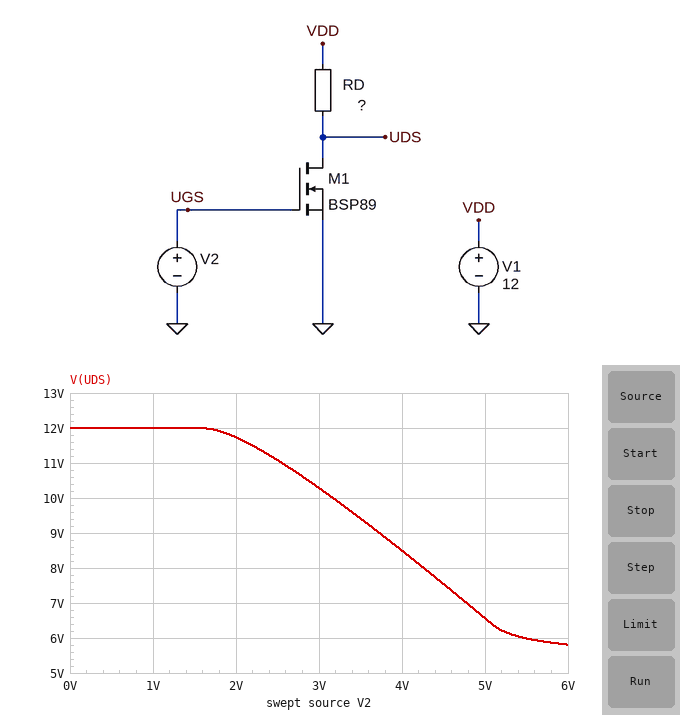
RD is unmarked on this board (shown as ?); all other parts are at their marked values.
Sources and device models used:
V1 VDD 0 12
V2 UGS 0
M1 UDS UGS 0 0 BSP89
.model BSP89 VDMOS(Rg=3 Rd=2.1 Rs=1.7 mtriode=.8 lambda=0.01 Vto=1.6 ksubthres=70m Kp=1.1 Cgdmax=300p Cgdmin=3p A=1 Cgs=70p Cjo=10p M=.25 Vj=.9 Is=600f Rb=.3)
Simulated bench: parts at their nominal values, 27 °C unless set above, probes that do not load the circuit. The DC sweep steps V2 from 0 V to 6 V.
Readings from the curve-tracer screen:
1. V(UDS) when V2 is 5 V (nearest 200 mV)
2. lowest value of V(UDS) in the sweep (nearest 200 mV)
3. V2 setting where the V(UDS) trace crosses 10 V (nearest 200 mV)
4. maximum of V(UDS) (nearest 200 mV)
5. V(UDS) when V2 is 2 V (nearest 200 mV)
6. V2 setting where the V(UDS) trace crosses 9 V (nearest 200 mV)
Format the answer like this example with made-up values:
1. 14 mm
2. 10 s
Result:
1. 6.6 V
2. 5.8 V
3. 3.2 V
4. 12.0 V
5. 11.8 V
6. 3.8 V
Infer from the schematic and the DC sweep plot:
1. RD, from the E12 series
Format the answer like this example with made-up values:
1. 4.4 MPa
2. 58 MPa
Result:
1. 4.7 Ω
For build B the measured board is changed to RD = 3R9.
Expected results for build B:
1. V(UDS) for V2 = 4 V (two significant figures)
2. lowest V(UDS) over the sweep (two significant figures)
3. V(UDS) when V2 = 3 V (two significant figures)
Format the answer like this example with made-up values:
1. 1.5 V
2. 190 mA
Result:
1. 9.1 V
2. 6.4 V
3. 11 V
